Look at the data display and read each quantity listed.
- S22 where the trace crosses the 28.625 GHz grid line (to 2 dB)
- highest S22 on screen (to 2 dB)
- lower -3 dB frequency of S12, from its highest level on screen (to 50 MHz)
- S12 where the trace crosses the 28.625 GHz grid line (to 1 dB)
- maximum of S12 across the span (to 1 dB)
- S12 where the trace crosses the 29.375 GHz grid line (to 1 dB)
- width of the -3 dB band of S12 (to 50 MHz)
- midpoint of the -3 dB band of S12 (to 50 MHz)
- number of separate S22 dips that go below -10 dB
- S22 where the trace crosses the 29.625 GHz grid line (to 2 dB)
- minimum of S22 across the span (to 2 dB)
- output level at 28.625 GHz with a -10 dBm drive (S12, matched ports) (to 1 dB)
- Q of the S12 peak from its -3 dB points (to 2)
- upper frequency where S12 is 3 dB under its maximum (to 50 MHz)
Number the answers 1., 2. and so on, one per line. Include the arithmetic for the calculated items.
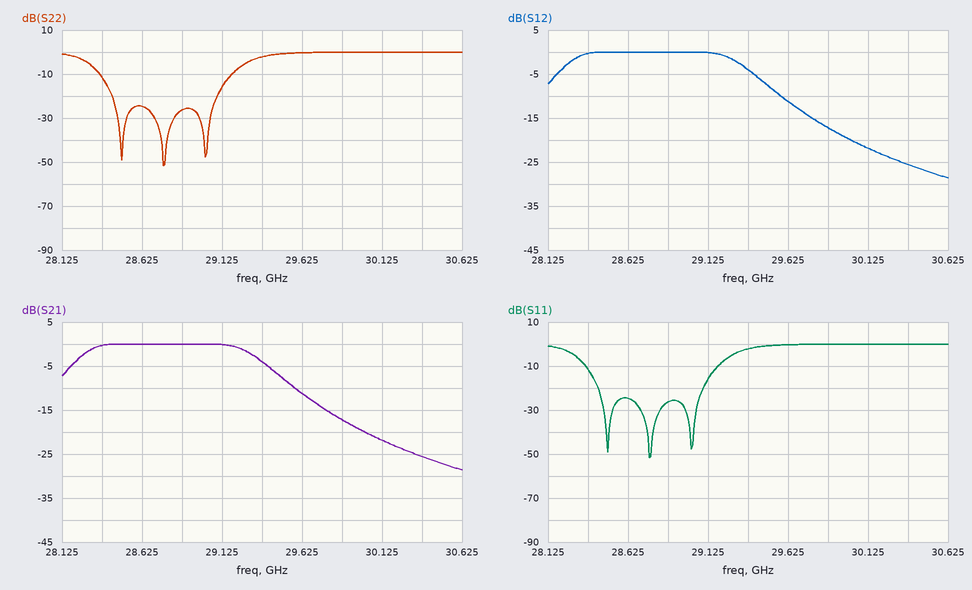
1. -24 dB
2. 0 dB
3. 28.25 GHz
4. 0 dB
5. 0 dB
6. -4 dB
7. 29.35 GHz − 28.25 GHz = 1.10 GHz
8. 28.80 GHz
9. 3
10. 0 dB
11. -52 dB
12. -10 dBm + (0 dB) = -10 dBm
13. 28.8 GHz / 1.1 GHz ≈ 26
14. 29.35 GHz
